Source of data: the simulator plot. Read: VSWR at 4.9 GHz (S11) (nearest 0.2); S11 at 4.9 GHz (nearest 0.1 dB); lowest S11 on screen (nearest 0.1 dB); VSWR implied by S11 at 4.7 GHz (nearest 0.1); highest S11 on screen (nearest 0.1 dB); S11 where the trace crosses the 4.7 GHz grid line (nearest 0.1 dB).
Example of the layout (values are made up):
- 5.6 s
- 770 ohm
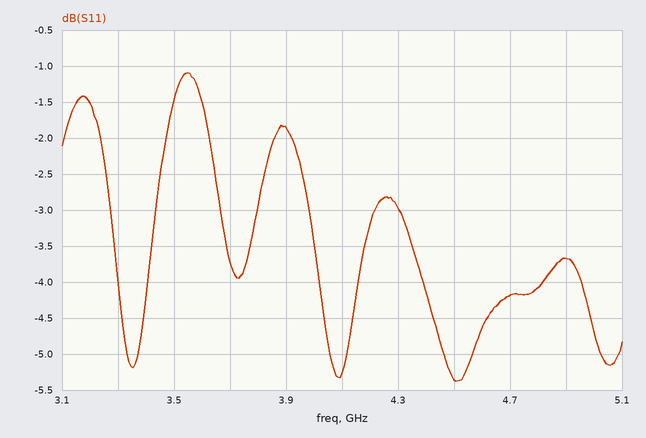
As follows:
- 4.8
- -3.7 dB
- -5.4 dB
- 4.2
- -1.1 dB
- -4.2 dB
